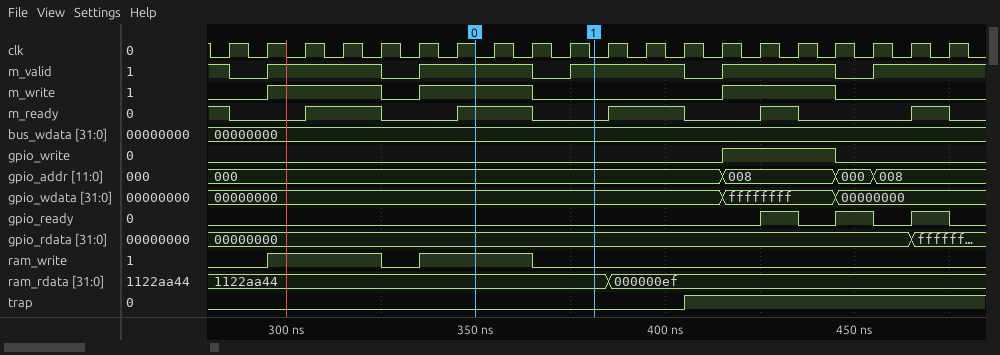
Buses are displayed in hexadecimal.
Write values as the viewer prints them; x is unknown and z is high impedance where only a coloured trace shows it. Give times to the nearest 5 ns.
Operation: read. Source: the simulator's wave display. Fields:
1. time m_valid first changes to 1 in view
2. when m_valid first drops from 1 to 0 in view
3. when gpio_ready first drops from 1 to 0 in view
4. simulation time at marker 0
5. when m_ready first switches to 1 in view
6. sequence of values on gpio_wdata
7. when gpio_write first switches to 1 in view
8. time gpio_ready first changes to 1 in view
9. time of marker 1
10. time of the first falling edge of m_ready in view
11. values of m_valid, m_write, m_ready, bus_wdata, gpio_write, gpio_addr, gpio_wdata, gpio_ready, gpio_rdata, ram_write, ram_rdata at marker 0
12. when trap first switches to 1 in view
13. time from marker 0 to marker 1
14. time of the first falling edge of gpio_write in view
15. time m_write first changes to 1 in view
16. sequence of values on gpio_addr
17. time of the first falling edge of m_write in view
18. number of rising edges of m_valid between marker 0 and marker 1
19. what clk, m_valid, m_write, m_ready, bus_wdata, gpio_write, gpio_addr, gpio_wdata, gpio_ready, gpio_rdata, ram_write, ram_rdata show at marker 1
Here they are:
295 ns
285 ns
435 ns
350 ns
305 ns
00000000, ffffffff, 00000000
415 ns
425 ns
380 ns
285 ns
m_valid=1, m_write=1, m_ready=1, bus_wdata=00000000, gpio_write=0, gpio_addr=000, gpio_wdata=00000000, gpio_ready=0, gpio_rdata=00000000, ram_write=1, ram_rdata=1122aa44
405 ns
30 ns
445 ns
295 ns
000, 008, 000, 008
325 ns
1
clk=0, m_valid=1, m_write=0, m_ready=0, bus_wdata=00000000, gpio_write=0, gpio_addr=000, gpio_wdata=00000000, gpio_ready=0, gpio_rdata=00000000, ram_write=0, ram_rdata=1122aa44
